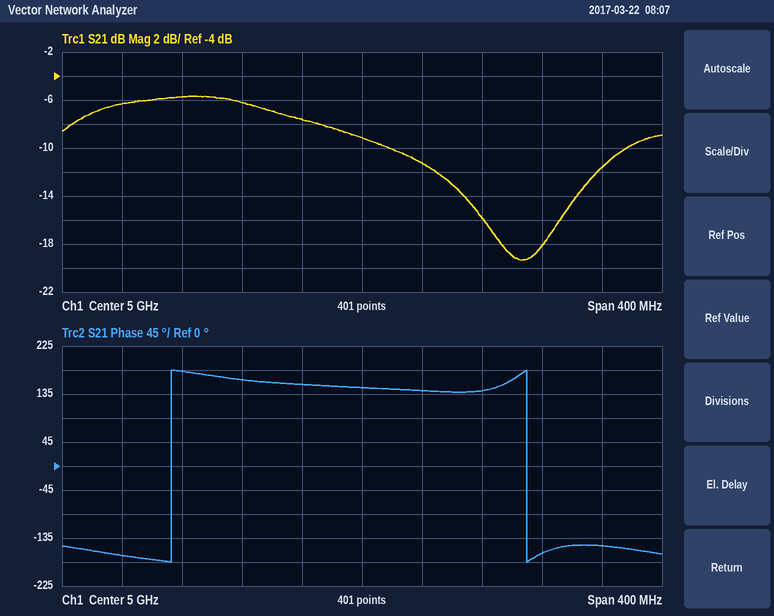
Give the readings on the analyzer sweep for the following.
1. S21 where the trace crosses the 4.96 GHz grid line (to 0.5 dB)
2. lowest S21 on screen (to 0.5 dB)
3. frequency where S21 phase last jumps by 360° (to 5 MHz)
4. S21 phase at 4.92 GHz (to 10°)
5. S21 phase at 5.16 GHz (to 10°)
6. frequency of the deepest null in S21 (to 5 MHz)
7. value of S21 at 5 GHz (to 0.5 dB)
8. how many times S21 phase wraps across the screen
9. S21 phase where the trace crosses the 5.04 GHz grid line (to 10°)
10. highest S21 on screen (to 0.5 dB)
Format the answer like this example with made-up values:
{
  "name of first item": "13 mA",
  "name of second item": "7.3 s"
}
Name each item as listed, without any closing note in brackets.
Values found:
{
  "S21 where the trace crosses the 4.96 GHz grid line": "-7.5 dB",
  "lowest S21 on screen": "-19.5 dB",
  "frequency where S21 phase last jumps by 360°": "5.110 GHz",
  "S21 phase at 4.92 GHz": "160°",
  "S21 phase at 5.16 GHz": "-150°",
  "frequency of the deepest null in S21": "5.105 GHz",
  "value of S21 at 5 GHz": "-9.0 dB",
  "how many times S21 phase wraps across the screen": "2",
  "S21 phase where the trace crosses the 5.04 GHz grid line": "140°",
  "highest S21 on screen": "-5.5 dB"
}
